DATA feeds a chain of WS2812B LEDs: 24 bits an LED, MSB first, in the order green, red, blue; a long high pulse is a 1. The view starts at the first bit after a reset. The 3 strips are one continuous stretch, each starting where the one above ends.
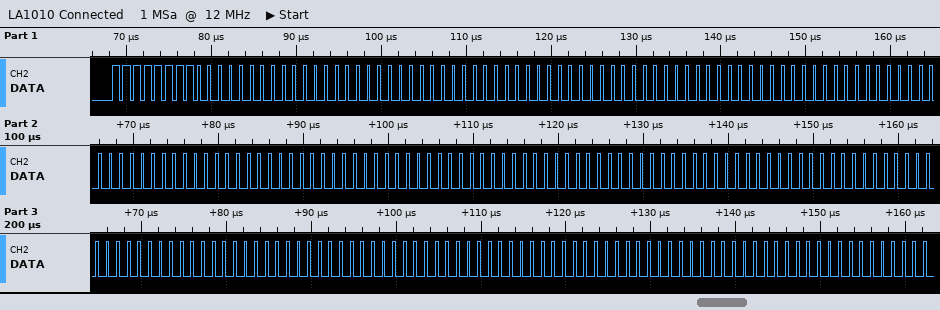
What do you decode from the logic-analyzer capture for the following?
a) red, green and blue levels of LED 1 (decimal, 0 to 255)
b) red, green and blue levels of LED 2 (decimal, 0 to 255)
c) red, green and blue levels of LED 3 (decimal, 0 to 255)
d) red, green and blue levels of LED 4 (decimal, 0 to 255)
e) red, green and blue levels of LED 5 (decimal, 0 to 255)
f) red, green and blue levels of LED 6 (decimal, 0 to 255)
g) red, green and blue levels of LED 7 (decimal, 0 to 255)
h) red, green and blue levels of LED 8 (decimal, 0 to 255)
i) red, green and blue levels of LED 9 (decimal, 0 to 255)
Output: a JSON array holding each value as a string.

["0, 255, 0", "0, 0, 0", "0, 0, 0", "0, 0, 0", "0, 0, 0", "0, 0, 0", "0, 0, 0", "0, 0, 0", "0, 0, 0"]
